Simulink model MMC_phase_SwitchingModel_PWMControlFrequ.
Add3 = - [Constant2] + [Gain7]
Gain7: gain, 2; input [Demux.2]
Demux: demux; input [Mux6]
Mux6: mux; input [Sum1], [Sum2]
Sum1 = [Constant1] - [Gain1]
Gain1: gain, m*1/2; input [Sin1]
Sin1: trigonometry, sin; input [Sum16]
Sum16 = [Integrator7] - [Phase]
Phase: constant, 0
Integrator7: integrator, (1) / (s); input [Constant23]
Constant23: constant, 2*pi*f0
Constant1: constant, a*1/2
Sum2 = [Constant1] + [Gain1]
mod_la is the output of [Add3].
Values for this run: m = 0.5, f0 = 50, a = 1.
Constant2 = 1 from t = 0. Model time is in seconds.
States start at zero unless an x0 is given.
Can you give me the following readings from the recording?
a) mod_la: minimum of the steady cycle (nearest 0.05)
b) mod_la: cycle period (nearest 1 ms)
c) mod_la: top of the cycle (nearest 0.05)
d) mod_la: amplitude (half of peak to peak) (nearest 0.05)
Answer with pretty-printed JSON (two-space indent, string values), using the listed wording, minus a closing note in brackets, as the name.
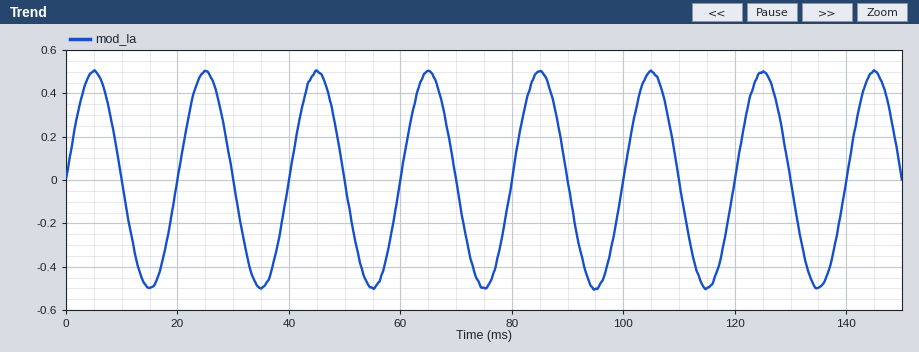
{
  "mod_la: minimum of the steady cycle": "-0.50",
  "mod_la: cycle period": "20 ms",
  "mod_la: top of the cycle": "0.50",
  "mod_la: amplitude (half of peak to peak)": "0.50"
}
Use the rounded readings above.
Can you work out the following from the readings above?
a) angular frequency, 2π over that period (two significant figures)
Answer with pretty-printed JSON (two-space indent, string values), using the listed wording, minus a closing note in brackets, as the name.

{
  "angular frequency, 2π over that period": "0.31 rad/ms"
}
